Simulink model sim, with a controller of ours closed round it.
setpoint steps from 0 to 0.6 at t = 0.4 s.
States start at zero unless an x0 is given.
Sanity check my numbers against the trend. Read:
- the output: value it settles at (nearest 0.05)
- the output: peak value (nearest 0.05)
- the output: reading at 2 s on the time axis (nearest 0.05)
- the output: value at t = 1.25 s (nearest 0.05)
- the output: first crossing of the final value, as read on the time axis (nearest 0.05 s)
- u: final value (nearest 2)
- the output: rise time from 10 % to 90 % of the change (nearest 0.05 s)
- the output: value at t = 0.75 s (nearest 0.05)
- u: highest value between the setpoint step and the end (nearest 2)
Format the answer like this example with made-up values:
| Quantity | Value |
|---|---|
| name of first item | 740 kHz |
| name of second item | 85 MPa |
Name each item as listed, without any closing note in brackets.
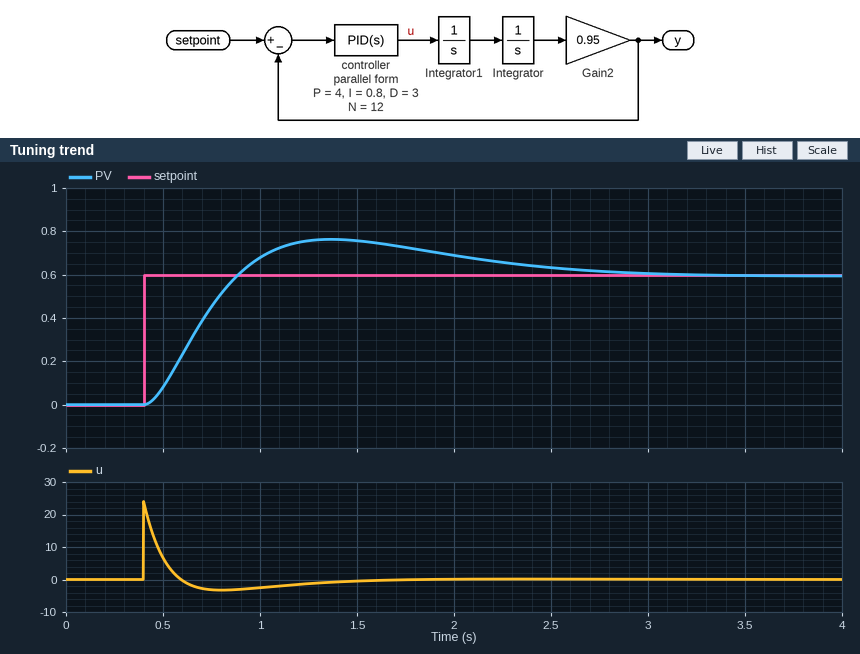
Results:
| Quantity | Value |
|---|---|
| the output: value it settles at | 0.60 |
| the output: peak value | 0.75 |
| the output: reading at 2 s on the time axis | 0.70 |
| the output: value at t = 1.25 s | 0.75 |
| the output: first crossing of the final value, as read on the time axis | 0.90 s |
| u: final value | 0 |
| the output: rise time from 10 % to 90 % of the change | 0.35 s |
| the output: value at t = 0.75 s | 0.45 |
| u: highest value between the setpoint step and the end | 24 |
